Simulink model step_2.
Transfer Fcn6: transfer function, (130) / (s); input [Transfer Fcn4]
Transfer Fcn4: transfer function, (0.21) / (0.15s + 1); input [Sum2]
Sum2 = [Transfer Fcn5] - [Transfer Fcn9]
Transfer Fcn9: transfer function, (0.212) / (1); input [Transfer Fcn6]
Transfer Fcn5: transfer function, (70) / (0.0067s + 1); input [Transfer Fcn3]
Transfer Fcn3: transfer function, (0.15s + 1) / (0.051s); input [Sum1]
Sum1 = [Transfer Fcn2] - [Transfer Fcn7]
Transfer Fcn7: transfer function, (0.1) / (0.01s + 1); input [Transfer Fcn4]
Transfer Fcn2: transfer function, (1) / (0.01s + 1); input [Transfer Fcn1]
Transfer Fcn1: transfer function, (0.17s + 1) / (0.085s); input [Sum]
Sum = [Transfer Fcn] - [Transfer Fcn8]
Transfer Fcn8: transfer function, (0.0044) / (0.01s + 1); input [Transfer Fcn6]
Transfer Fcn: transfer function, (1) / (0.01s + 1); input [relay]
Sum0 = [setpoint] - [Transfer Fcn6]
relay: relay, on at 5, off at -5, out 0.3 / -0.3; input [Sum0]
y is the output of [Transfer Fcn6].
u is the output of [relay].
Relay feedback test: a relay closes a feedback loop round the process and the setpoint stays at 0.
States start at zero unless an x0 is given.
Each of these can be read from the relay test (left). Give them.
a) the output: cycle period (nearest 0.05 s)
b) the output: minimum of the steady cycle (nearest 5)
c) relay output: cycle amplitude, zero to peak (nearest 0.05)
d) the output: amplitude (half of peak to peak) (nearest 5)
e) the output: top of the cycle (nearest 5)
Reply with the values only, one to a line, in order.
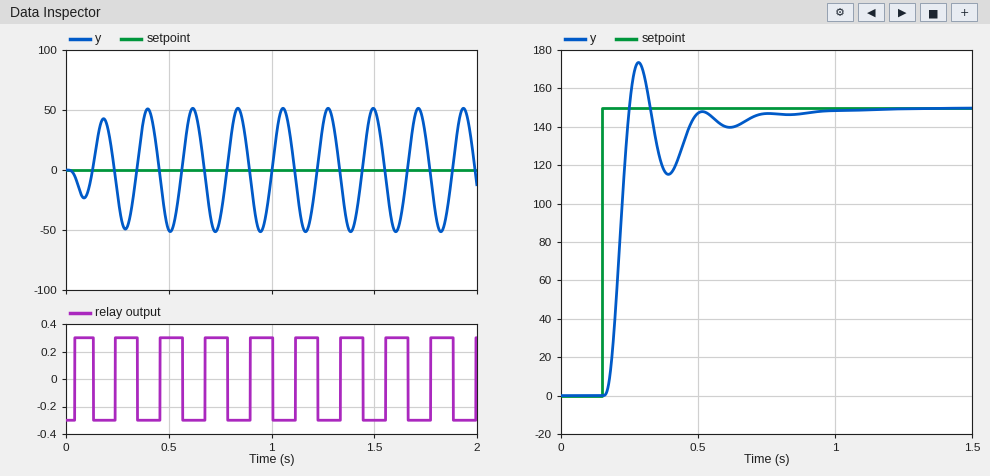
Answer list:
0.20 s
-50
0.30
50
50
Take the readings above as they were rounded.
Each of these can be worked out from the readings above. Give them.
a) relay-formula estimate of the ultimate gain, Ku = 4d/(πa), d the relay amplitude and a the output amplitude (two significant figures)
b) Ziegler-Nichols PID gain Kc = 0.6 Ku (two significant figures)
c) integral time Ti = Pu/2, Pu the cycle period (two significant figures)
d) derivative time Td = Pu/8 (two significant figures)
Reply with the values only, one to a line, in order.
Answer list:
0.0076
0.0046
0.10 s
0.025 s
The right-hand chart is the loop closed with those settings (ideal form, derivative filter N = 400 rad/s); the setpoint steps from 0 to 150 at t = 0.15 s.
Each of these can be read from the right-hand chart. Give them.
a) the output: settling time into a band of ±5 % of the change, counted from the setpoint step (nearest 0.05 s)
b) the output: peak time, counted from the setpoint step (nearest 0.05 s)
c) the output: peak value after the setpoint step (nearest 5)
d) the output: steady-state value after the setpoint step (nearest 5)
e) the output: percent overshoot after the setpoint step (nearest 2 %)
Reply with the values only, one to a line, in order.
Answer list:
0.50 s
0.15 s
175
150
16 %
